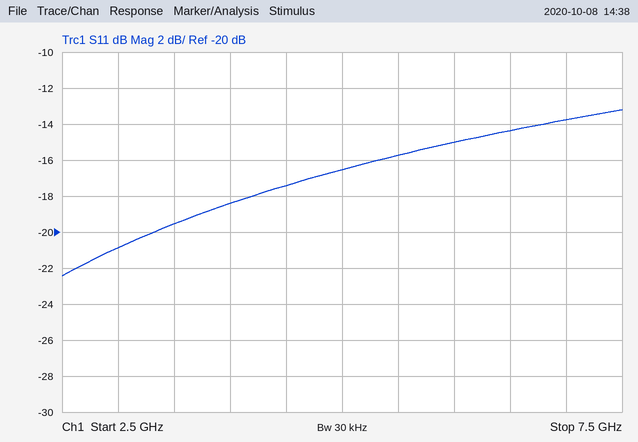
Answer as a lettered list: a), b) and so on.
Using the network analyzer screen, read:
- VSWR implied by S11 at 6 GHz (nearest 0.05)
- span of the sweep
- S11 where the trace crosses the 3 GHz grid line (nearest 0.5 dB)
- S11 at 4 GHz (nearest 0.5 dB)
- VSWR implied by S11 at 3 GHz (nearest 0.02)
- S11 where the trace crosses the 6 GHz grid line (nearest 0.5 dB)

a) 1.45
b) 5 GHz
c) -21.0 dB
d) -18.5 dB
e) 1.20
f) -15.0 dB
